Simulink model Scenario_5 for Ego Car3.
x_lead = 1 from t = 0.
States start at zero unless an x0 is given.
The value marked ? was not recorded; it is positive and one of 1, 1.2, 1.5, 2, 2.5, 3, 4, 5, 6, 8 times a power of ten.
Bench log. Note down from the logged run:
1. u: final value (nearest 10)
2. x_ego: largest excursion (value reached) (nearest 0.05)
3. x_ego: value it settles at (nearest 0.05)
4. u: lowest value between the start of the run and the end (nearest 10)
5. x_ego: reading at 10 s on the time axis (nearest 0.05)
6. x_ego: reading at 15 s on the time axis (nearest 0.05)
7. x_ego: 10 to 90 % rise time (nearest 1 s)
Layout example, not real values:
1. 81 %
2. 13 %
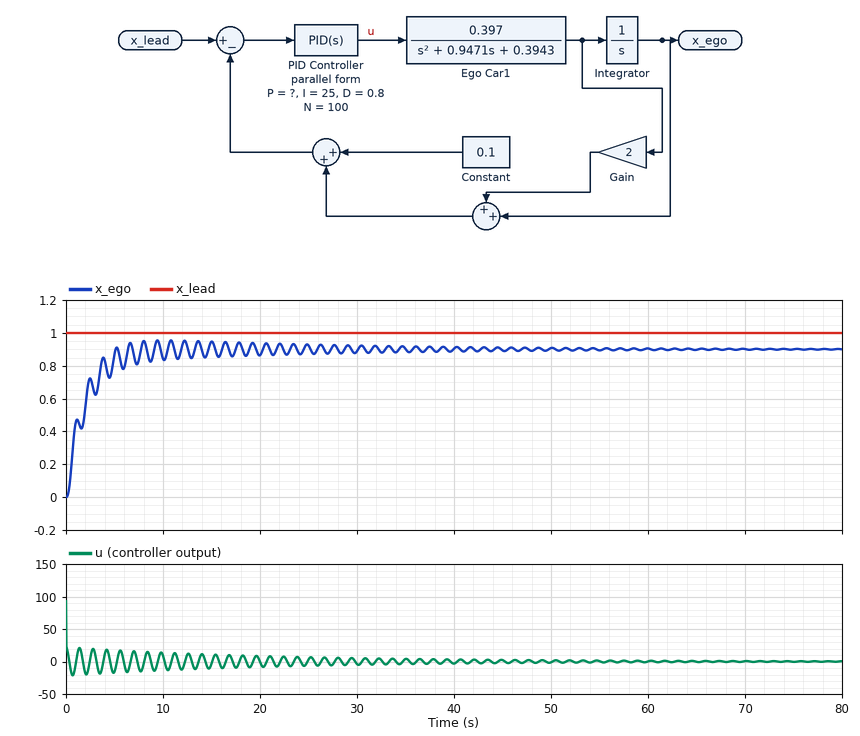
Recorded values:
1. 0
2. 0.95
3. 0.90
4. -20
5. 0.85
6. 0.95
7. 3 s
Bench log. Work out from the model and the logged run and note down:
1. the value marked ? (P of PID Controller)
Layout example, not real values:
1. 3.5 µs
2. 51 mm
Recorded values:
1. 25
